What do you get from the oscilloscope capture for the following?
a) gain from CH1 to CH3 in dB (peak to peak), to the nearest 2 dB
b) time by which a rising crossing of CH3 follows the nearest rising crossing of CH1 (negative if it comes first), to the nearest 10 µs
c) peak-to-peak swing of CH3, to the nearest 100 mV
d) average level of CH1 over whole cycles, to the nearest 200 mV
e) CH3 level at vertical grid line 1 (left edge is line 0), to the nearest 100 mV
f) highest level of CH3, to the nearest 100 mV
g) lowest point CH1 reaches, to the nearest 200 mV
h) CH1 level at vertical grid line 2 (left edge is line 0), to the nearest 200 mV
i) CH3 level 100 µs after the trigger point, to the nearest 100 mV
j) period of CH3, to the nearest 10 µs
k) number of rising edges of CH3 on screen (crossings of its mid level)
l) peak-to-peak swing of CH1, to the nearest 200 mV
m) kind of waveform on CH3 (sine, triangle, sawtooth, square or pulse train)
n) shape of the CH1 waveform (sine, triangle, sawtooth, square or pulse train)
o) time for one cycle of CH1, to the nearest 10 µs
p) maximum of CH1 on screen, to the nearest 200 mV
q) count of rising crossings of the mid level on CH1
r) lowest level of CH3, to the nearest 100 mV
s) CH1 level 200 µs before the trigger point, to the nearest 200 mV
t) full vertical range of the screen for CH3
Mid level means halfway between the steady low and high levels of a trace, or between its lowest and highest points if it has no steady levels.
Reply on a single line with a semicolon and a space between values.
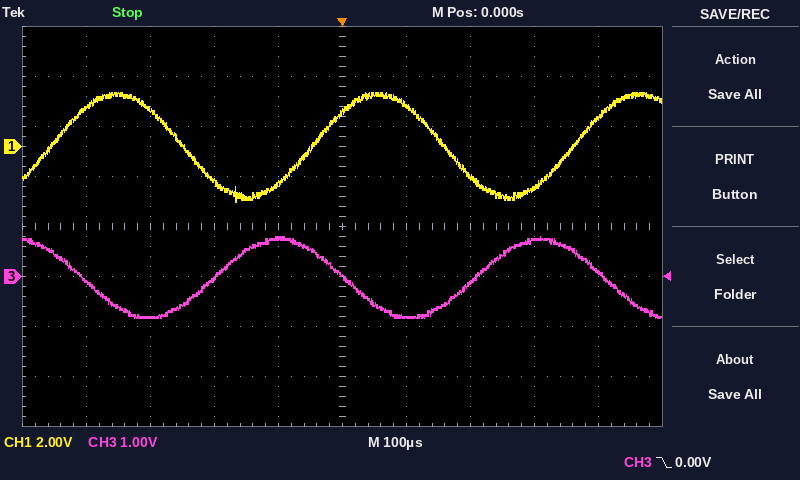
-8 dB; -150 µs; 1.6 V; 0.0 V; -100 mV; 800 mV; -2.2 V; 1.4 V; -800 mV; 410 µs; 2; 4.4 V; sine; sine; 410 µs; 2.2 V; 3; -800 mV; -1.4 V; 8 V
